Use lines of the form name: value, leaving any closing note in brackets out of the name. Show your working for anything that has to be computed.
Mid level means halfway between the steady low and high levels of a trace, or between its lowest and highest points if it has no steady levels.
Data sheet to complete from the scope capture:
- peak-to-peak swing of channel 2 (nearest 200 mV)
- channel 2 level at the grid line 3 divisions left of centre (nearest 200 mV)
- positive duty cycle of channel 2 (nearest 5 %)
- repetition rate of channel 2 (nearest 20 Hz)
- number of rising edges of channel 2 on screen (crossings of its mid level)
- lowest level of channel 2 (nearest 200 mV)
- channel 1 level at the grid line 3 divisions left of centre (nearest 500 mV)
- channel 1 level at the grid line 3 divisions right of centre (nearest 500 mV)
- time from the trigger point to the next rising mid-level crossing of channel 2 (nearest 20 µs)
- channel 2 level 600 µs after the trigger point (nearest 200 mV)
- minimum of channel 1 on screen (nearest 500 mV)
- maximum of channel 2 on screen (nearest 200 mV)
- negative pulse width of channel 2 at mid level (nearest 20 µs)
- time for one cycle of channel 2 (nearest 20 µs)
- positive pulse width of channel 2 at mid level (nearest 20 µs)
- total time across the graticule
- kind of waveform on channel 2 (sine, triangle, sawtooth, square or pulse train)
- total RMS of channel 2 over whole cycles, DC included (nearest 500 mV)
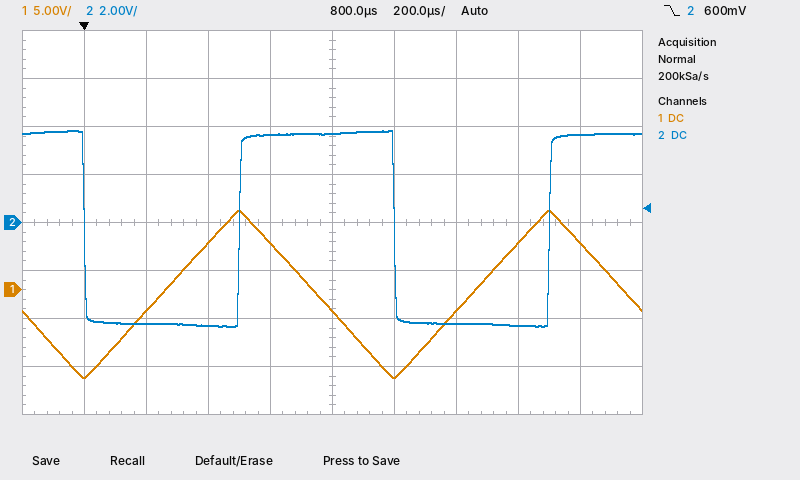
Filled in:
peak-to-peak swing of channel 2: 3.8 V − (-4.4 V) = 8.2 V
channel 2 level at the grid line 3 divisions left of centre: -4.2 V
positive duty cycle of channel 2: 500 µs / 1.00 ms ≈ 50 %
repetition rate of channel 2: 1 / 1.00 ms ≈ 1.00 kHz
number of rising edges of channel 2 on screen: 2
lowest level of channel 2: -4.4 V
channel 1 level at the grid line 3 divisions left of centre: -2.0 V
channel 1 level at the grid line 3 divisions right of centre: 5.0 V
time from the trigger point to the next rising mid-level crossing of channel 2: 500 µs
channel 2 level 600 µs after the trigger point: 3.6 V
minimum of channel 1 on screen: -9.0 V
maximum of channel 2 on screen: 3.8 V
negative pulse width of channel 2 at mid level: 500 µs
time for one cycle of channel 2: 1.00 ms
positive pulse width of channel 2 at mid level: 500 µs
total time across the graticule: 2 ms
kind of waveform on channel 2: square
total RMS of channel 2 over whole cycles, DC included: √(0.5 × (3.8 V)² + 0.5 × (-4.4 V)²) ≈ 4.11 V, so 4.0 V to the nearest 500 mV
